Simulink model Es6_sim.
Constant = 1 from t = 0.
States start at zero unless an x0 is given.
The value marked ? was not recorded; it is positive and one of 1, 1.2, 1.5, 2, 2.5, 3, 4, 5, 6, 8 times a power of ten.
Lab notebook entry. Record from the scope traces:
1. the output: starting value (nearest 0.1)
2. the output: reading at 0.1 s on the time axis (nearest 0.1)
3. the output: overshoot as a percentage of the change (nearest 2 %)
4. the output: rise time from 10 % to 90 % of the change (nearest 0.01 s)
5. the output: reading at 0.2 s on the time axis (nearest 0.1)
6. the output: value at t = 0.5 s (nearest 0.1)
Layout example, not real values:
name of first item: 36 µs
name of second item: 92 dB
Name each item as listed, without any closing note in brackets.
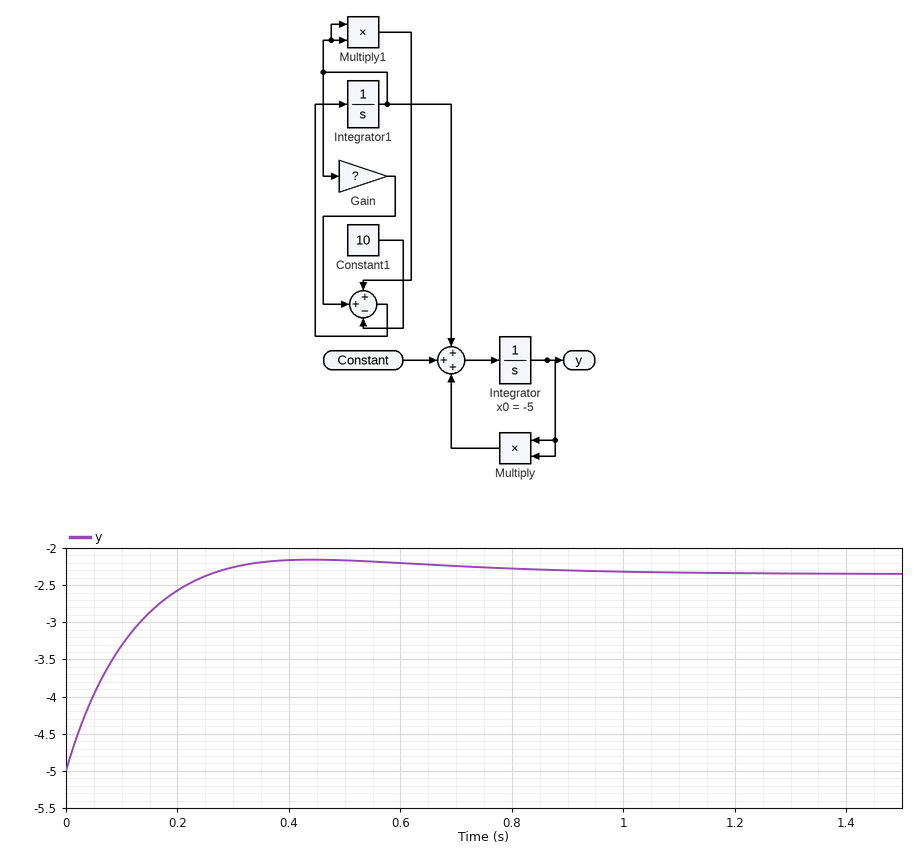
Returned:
the output: starting value: -5.0
the output: reading at 0.1 s on the time axis: -3.3
the output: overshoot as a percentage of the change: 8 %
the output: rise time from 10 % to 90 % of the change: 0.18 s
the output: reading at 0.2 s on the time axis: -2.6
the output: value at t = 0.5 s: -2.2
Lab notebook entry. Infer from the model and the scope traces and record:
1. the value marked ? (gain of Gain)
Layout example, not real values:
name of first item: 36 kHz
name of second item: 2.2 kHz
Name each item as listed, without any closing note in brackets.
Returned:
the value marked ?: 5
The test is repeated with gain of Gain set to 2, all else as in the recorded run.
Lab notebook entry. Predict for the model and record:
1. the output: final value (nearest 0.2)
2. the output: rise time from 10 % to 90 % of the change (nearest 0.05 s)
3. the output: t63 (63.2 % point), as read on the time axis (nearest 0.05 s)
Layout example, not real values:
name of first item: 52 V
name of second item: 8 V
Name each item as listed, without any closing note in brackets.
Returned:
the output: final value: -1.8
the output: rise time from 10 % to 90 % of the change: 0.30 s
the output: t63 (63.2 % point), as read on the time axis: 0.15 s
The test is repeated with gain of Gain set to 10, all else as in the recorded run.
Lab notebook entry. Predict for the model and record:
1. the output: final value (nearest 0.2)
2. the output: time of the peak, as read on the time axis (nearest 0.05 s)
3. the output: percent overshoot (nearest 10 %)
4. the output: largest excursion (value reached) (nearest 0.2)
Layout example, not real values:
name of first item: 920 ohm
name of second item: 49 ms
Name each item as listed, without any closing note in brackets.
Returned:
the output: final value: -3.2
the output: time of the peak, as read on the time axis: 0.30 s
the output: percent overshoot: 30 %
the output: largest excursion (value reached): -2.6
